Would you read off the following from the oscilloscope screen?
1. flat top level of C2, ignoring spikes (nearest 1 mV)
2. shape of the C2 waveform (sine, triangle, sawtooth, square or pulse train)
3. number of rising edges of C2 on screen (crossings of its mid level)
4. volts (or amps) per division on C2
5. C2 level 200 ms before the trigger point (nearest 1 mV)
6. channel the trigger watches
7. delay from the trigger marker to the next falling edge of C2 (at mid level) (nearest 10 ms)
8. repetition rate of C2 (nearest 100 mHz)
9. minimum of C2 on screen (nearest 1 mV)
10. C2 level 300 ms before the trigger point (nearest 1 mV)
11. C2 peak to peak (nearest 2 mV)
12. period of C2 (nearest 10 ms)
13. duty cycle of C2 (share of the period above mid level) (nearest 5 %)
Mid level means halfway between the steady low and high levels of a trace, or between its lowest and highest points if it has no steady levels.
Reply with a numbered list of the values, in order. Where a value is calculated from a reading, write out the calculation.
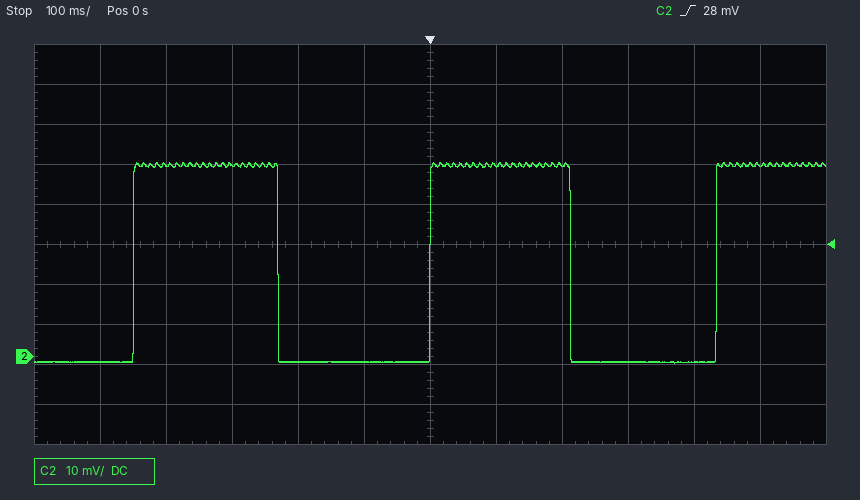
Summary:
1. 48 mV
2. square
3. 3
4. 10 mV
5. -1 mV
6. C2
7. 210 ms
8. 1 / 440 ms ≈ 2.3 Hz
9. -2 mV
10. 48 mV
11. 50 mV
12. 440 ms
13. 50 %
